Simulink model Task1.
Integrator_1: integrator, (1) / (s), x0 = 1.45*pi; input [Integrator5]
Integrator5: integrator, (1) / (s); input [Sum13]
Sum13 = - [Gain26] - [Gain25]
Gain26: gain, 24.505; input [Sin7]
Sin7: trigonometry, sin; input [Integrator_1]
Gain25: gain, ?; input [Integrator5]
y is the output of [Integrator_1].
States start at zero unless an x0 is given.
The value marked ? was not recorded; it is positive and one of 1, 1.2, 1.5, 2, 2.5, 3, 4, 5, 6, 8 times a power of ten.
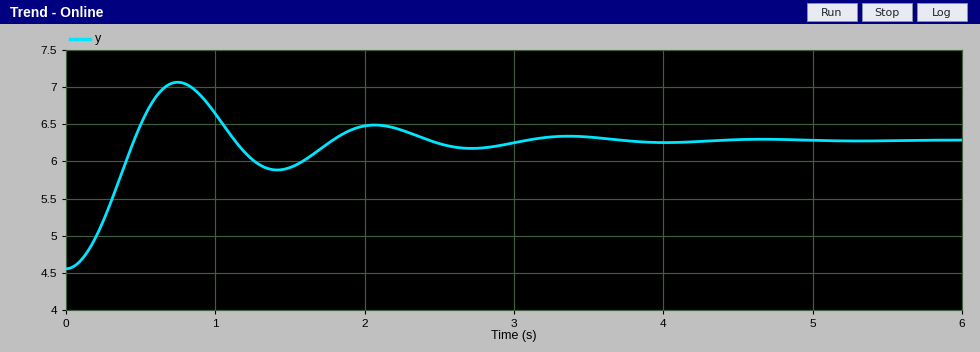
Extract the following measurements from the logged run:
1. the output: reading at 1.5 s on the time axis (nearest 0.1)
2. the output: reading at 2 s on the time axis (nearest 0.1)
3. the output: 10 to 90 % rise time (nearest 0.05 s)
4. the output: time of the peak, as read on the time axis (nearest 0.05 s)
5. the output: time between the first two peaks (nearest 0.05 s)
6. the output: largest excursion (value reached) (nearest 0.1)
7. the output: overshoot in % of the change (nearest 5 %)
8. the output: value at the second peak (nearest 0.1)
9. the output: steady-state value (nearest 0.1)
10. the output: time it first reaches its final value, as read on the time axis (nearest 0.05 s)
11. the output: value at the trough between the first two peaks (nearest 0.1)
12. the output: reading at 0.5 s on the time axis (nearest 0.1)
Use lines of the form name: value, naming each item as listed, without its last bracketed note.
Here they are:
the output: reading at 1.5 s on the time axis: 5.9
the output: reading at 2 s on the time axis: 6.5
the output: 10 to 90 % rise time: 0.30 s
the output: time of the peak, as read on the time axis: 0.75 s
the output: time between the first two peaks: 1.30 s
the output: largest excursion (value reached): 7.1
the output: overshoot in % of the change: 45 %
the output: value at the second peak: 6.5
the output: steady-state value: 6.3
the output: time it first reaches its final value, as read on the time axis: 0.45 s
the output: value at the trough between the first two peaks: 5.9
the output: reading at 0.5 s on the time axis: 6.5
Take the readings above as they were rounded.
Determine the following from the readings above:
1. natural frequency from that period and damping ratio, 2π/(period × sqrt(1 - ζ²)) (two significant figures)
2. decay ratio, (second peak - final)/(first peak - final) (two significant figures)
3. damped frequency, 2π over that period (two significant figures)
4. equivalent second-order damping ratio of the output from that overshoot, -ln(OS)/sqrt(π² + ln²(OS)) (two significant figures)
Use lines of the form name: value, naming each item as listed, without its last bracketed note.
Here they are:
natural frequency from that period and damping ratio, 2π/(period × sqrt(1 - ζ²)): 5.0 rad/s
decay ratio, (second peak - final)/(first peak - final): 0.25
damped frequency, 2π over that period: 4.8 rad/s
equivalent second-order damping ratio of the output from that overshoot, -ln(OS)/sqrt(π² + ln²(OS)): 0.25
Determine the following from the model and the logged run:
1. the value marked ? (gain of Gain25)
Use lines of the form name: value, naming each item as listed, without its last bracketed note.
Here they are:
the value marked ?: 2
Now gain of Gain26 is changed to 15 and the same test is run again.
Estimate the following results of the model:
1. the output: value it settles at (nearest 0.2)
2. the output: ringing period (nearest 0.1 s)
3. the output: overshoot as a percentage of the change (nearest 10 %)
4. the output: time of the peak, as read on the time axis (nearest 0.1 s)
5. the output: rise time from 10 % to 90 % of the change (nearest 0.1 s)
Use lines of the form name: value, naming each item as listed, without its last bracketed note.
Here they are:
the output: value it settles at: 6.2
the output: ringing period: 1.7 s
the output: overshoot as a percentage of the change: 40 %
the output: time of the peak, as read on the time axis: 1.0 s
the output: rise time from 10 % to 90 % of the change: 0.4 s
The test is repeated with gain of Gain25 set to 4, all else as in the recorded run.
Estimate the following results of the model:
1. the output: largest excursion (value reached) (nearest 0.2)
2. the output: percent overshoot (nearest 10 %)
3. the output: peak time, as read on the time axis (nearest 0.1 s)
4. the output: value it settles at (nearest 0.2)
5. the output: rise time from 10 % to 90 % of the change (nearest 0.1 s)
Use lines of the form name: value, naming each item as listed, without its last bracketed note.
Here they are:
the output: largest excursion (value reached): 6.6
the output: percent overshoot: 20 %
the output: peak time, as read on the time axis: 0.8 s
the output: value it settles at: 6.2
the output: rise time from 10 % to 90 % of the change: 0.4 s
